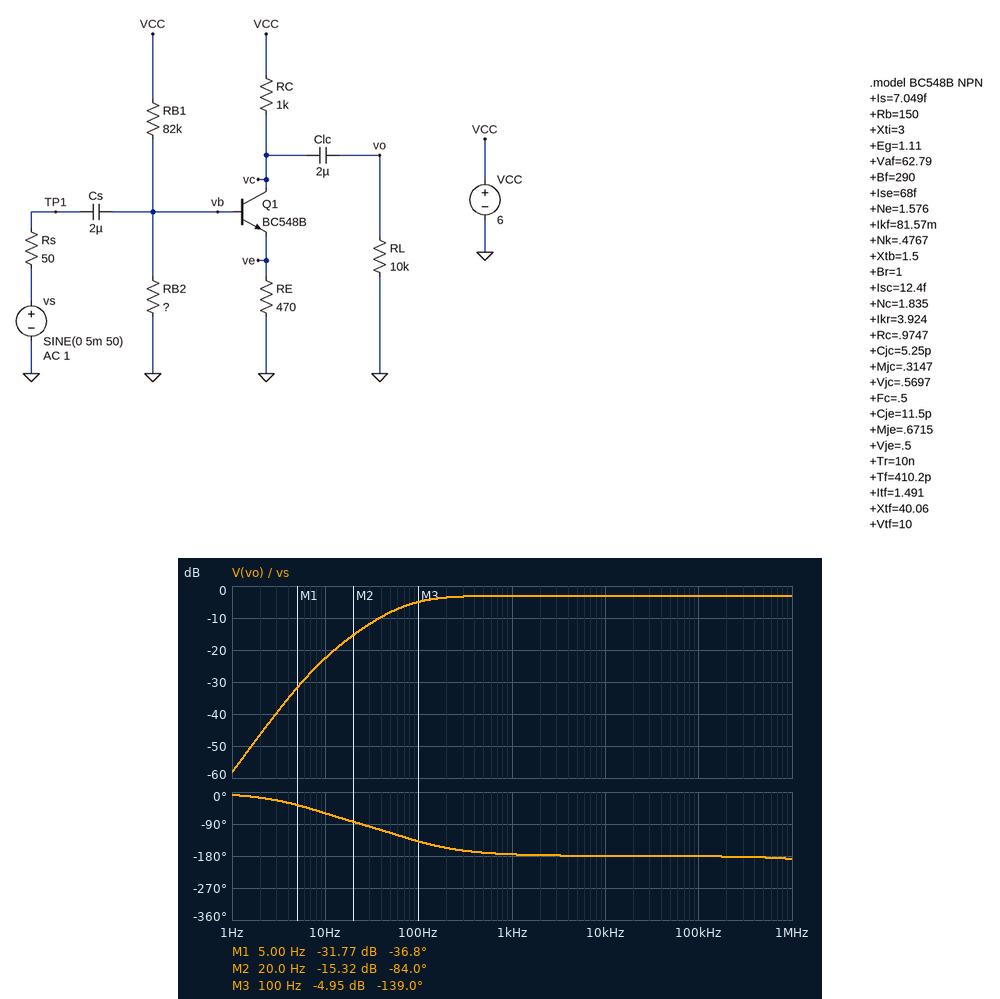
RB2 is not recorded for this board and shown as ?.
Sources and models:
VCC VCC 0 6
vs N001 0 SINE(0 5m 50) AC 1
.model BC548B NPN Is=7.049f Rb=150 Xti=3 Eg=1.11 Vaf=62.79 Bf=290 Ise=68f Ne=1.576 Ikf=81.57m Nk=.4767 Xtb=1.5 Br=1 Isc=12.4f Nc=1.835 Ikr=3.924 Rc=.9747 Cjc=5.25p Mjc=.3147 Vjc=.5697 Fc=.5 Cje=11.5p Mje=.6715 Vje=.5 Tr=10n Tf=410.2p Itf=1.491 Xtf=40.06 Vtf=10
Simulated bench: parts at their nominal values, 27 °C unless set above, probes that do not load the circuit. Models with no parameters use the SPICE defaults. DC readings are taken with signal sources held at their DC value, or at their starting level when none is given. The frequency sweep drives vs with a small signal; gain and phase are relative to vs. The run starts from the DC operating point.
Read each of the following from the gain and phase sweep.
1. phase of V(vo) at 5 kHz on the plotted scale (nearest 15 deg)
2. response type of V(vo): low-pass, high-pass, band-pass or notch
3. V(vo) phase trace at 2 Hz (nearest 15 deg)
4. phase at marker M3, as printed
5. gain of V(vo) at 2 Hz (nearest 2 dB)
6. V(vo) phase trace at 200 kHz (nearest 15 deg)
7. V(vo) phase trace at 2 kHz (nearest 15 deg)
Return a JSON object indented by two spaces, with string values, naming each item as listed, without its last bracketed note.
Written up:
{
  "phase of V(vo) at 5 kHz on the plotted scale": "-180 deg",
  "response type of V(vo): low-pass, high-pass, band-pass or notch": "high-pass",
  "V(vo) phase trace at 2 Hz": "-15 deg",
  "phase at marker M3, as printed": "-139.0 deg",
  "gain of V(vo) at 2 Hz": "-46 dB",
  "V(vo) phase trace at 200 kHz": "-180 deg",
  "V(vo) phase trace at 2 kHz": "-180 deg"
}
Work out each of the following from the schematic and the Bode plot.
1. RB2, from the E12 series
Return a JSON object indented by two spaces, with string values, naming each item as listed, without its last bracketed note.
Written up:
{
  "RB2, from the E12 series": "270 kΩ"
}
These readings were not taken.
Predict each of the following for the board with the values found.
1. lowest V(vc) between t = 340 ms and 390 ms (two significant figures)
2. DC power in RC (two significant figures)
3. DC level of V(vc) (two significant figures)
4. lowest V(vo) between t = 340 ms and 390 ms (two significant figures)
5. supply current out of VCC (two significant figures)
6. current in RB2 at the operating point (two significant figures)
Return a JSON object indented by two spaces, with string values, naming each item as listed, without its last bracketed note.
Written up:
{
  "lowest V(vc) between t = 340 ms and 390 ms": "2.0 V",
  "DC power in RC": "16 mW",
  "DC level of V(vc)": "2.0 V",
  "lowest V(vo) between t = 340 ms and 390 ms": "-1.9 mV",
  "supply current out of VCC": "4.0 mA",
  "current in RB2 at the operating point": "9.6 µA"
}
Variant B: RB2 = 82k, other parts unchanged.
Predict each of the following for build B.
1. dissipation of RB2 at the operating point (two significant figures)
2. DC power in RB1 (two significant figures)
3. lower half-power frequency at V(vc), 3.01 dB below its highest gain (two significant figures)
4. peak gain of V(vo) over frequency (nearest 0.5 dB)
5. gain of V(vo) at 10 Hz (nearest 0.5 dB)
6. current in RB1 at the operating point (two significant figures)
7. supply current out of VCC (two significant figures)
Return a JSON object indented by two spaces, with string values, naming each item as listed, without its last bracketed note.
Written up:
{
  "dissipation of RB2 at the operating point": "70 µW",
  "DC power in RB1": "160 µW",
  "lower half-power frequency at V(vc), 3.01 dB below its highest gain": "2.3 Hz",
  "peak gain of V(vo) over frequency": "5.5 dB",
  "gain of V(vo) at 10 Hz": "3.5 dB",
  "current in RB1 at the operating point": "44 µA",
  "supply current out of VCC": "3.6 mA"
}
